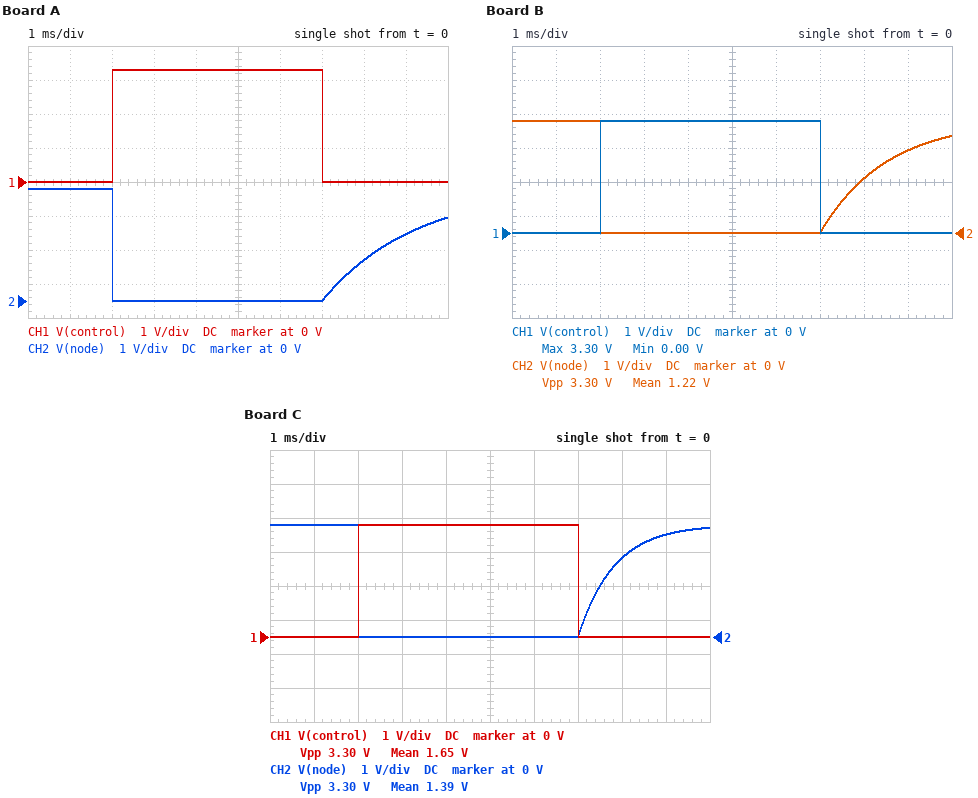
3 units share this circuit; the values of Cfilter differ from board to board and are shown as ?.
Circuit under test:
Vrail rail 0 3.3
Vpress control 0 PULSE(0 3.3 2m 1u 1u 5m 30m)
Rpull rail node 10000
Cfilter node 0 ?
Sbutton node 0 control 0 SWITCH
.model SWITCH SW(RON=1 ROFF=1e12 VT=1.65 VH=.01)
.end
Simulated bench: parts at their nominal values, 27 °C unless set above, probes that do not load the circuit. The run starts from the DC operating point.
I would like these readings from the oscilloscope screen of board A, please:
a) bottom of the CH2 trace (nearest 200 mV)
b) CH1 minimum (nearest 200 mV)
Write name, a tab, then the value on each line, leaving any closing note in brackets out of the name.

bottom of the CH2 trace	0 V
CH1 minimum	0 V
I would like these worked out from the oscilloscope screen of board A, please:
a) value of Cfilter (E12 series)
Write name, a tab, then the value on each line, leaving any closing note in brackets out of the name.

value of Cfilter	220 nF
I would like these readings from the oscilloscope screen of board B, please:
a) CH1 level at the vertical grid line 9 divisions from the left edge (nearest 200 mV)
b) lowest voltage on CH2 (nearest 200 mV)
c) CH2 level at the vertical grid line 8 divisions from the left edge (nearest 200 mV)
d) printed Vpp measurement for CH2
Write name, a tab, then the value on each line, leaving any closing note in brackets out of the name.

CH1 level at the vertical grid line 9 divisions from the left edge	0 V
lowest voltage on CH2	0 V
CH2 level at the vertical grid line 8 divisions from the left edge	1.6 V
printed Vpp measurement for CH2	3.30 V
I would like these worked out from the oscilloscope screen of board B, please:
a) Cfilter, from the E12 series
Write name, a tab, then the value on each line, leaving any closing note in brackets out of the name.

Cfilter, from the E12 series	150 nF
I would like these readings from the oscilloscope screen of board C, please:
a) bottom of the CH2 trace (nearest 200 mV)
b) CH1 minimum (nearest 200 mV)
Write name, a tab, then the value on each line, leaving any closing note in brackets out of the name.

bottom of the CH2 trace	0 V
CH1 minimum	0 V
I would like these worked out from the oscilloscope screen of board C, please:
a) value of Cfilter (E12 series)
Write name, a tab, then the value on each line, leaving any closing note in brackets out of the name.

value of Cfilter	82 nF
